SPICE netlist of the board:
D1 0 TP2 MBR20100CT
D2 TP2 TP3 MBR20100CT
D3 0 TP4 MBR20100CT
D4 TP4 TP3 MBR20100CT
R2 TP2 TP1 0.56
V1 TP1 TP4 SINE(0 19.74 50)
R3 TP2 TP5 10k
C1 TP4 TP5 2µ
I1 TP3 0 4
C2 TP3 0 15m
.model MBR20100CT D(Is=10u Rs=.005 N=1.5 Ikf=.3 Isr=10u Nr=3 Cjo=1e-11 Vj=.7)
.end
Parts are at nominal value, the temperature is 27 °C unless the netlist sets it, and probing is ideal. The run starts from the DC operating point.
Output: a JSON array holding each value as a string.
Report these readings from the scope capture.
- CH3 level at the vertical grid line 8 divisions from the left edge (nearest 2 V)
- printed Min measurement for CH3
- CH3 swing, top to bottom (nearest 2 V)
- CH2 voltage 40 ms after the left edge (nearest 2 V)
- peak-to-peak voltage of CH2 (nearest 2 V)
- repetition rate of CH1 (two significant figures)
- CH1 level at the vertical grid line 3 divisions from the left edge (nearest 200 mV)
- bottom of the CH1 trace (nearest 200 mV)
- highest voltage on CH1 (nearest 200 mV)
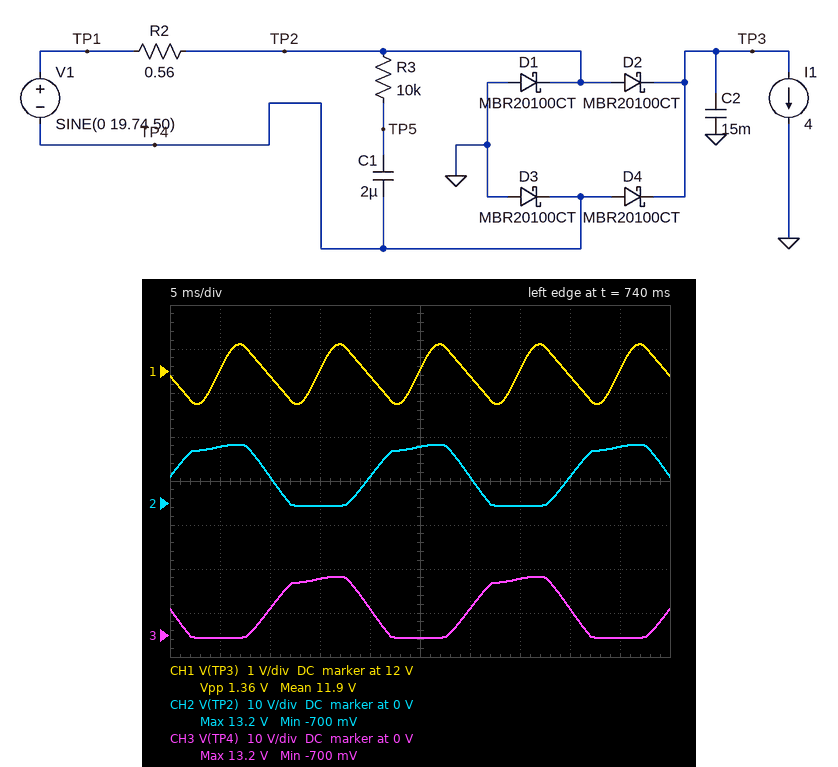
["6 V", "-700 mV", "14 V", "6 V", "14 V", "100 Hz", "12.0 V", "11.2 V", "12.6 V"]
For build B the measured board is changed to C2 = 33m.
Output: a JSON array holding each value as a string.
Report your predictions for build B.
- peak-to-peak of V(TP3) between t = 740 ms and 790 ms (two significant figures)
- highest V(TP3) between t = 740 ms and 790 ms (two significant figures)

["620 mV", "12 V"]
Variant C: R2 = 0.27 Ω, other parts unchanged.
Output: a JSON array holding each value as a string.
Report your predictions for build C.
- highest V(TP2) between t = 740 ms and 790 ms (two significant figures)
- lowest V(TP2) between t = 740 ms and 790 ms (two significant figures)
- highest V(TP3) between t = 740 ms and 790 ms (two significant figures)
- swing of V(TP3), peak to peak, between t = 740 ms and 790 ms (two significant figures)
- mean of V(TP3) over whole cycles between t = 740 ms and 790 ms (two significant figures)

["16 V", "-770 mV", "15 V", "1.6 V", "14 V"]
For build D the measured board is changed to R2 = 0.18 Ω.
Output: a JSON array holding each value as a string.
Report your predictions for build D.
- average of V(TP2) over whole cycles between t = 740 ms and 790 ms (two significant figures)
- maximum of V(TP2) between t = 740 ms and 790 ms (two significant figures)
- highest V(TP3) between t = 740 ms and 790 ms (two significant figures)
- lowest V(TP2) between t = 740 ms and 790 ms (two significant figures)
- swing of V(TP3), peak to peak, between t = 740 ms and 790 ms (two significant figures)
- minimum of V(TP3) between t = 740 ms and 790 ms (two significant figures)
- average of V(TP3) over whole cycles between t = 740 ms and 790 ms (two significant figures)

["7.6 V", "17 V", "16 V", "-790 mV", "1.7 V", "14 V", "15 V"]
